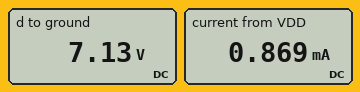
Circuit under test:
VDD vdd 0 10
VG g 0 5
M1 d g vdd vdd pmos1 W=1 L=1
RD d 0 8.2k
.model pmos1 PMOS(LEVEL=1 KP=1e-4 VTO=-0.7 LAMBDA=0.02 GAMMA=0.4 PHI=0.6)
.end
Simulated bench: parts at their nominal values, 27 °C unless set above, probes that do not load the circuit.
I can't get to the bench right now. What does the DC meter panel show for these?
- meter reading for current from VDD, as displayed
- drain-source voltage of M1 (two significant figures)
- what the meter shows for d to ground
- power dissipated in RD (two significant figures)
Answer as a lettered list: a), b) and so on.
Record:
a) 0.869 mA
b) -2.9 V
c) 7.13 V
d) 6.2 mW
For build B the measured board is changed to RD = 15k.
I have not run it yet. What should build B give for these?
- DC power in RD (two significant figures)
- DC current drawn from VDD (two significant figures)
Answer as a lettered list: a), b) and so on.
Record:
a) 4.8 mW
b) 560 µA
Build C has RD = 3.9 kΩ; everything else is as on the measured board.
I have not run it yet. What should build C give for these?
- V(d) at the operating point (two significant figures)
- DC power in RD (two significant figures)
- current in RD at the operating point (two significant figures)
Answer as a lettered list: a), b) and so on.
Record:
a) 4.0 V
b) 4.2 mW
c) 1.0 mA
